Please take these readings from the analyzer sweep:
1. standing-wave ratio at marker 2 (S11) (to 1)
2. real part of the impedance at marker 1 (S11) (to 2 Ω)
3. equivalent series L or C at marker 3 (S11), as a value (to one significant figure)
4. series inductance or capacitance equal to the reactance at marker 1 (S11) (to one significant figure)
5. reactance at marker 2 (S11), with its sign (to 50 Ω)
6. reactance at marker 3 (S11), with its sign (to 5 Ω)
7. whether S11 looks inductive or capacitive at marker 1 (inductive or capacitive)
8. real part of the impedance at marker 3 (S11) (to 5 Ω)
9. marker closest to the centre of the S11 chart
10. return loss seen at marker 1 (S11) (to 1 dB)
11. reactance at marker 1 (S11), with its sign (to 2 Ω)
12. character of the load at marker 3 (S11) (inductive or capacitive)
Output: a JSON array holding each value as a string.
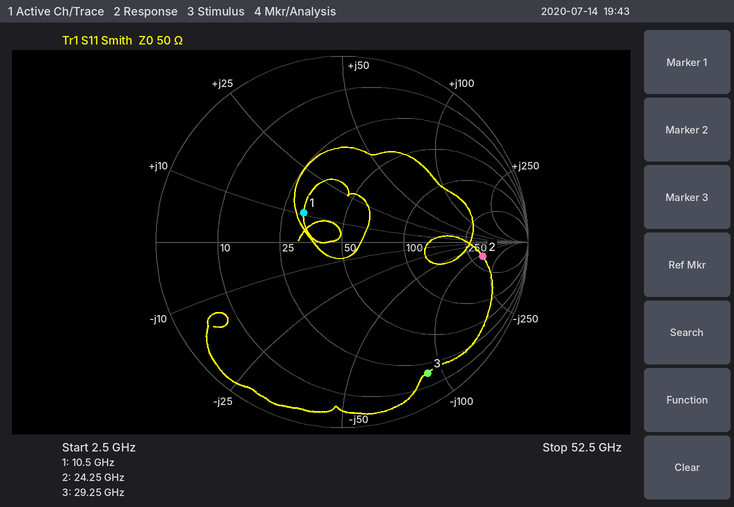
["7", "32 Ω", "60 fF", "200 pH", "-100 Ω", "-90 Ω", "inductive", "20 Ω", "marker 1", "12 dB", "+10 Ω", "capacitive"]
